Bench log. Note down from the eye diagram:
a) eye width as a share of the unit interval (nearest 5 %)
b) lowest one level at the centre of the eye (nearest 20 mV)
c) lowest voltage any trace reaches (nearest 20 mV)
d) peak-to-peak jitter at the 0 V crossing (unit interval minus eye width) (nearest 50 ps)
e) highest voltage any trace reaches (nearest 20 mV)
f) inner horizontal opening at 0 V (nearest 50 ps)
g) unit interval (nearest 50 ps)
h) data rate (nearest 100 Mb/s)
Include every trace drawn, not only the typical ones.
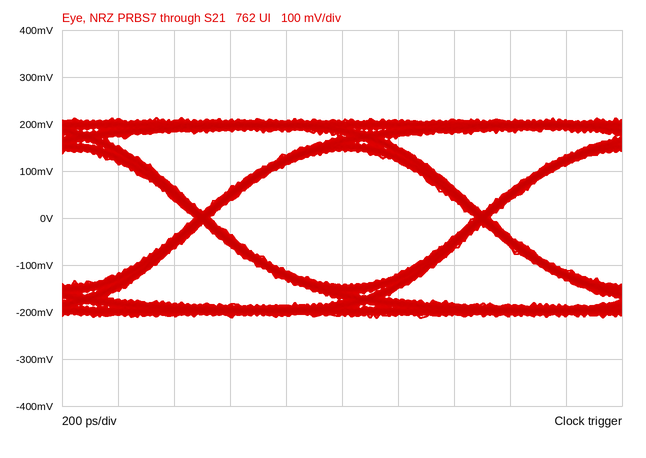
95 %
140 mV
-220 mV
50 ps
220 mV
950 ps
1.00 ns
1.0 Gb/s
